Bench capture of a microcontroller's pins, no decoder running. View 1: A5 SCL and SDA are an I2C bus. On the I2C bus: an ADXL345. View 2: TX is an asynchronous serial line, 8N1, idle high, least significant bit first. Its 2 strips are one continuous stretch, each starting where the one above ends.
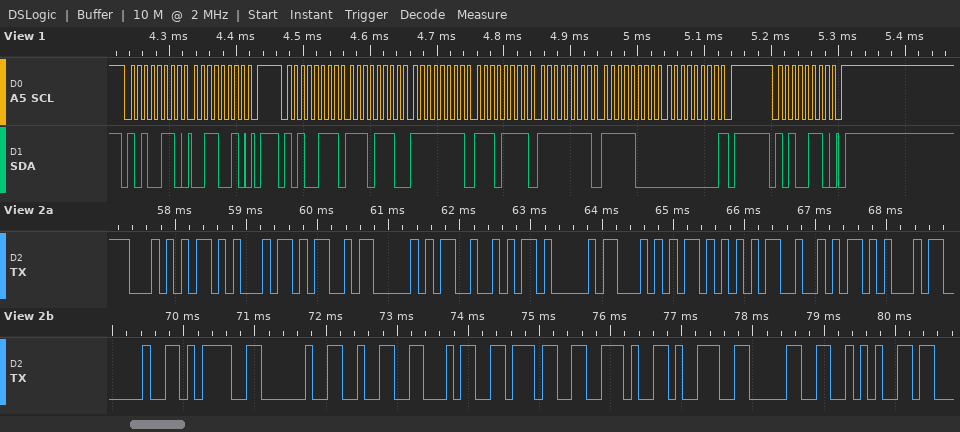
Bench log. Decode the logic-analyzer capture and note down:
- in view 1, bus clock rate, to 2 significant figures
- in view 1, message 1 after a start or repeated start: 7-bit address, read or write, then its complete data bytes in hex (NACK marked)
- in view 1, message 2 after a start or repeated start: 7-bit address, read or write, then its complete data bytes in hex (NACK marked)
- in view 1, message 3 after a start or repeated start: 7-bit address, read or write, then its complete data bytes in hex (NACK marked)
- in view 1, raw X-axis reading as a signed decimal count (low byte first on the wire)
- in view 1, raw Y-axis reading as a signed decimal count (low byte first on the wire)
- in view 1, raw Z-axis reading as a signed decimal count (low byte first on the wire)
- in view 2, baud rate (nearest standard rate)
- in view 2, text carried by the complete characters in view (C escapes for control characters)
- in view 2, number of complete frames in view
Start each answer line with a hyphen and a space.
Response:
- 100 kHz
- 0x53 write: 32
- 0x53 read: EE FF EF FF F8 00 NACK
- 0x53 write
- -18
- -17
- 248
- 9600 baud
- "TEMPRATURE = 247.90*"
- 20
